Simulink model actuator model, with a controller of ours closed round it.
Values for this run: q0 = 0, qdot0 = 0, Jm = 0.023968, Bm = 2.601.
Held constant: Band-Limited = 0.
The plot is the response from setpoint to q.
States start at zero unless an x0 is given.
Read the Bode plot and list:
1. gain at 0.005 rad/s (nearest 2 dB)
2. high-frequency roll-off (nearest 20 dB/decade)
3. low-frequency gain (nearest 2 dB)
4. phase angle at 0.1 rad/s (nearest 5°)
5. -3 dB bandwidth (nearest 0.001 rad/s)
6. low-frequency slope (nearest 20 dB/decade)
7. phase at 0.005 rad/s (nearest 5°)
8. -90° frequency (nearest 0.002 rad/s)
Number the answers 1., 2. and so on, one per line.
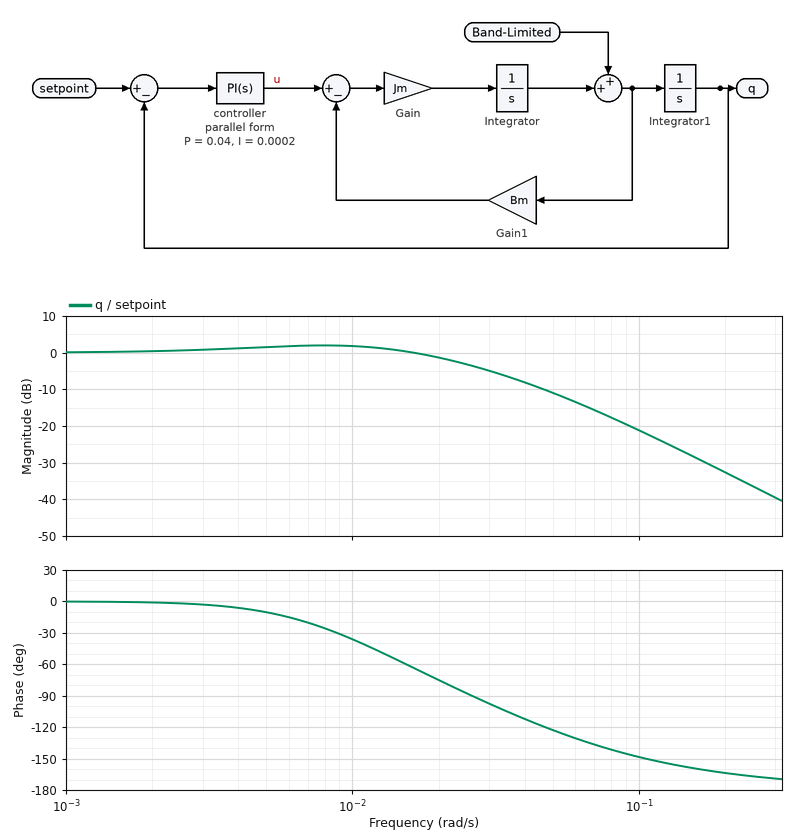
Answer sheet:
1. 2 dB
2. -40 dB/decade
3. 0 dB
4. -150°
5. 0.024 rad/s
6. 0 dB/decade
7. -10°
8. 0.026 rad/s
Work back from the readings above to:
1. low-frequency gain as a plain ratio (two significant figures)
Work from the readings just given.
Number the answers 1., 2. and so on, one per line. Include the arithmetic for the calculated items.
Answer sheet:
1. 10^(0 / 20) = 1.0
